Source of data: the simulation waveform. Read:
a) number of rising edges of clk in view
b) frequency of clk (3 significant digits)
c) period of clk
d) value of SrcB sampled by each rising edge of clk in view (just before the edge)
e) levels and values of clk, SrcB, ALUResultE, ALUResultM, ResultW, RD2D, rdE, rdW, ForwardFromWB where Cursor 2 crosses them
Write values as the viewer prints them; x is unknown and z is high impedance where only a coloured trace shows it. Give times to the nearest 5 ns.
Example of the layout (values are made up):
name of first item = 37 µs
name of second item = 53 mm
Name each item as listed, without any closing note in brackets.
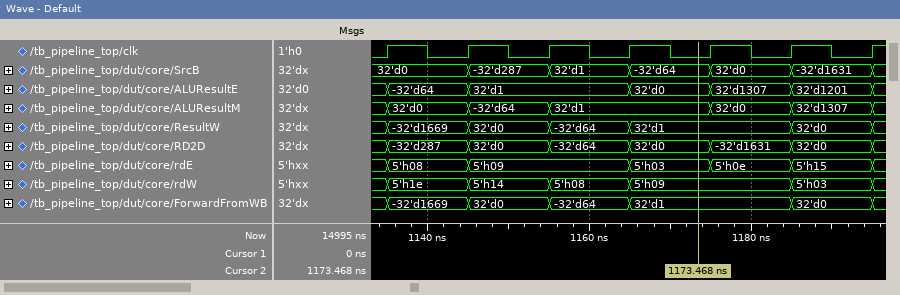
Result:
number of rising edges of clk in view = 7
frequency of clk = 100 MHz
period of clk = 10 ns
value of SrcB sampled by each rising edge of clk in view = 32'd0, 32'd0, -32'd287, 32'd1, -32'd64, 32'd0, -32'd1631
levels and values of clk, SrcB, ALUResultE, ALUResultM, ResultW, RD2D, rdE, rdW, ForwardFromWB where Cursor 2 crosses them = clk=0, SrcB=-32'd64, ALUResultE=32'd0, ALUResultM=32'd1, ResultW=32'd1, RD2D=32'd0, rdE=5'h03, rdW=5'h09, ForwardFromWB=32'd1
